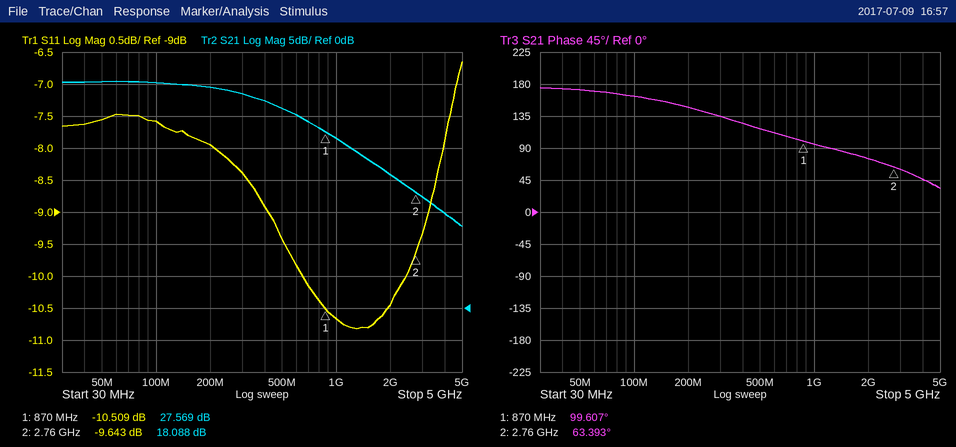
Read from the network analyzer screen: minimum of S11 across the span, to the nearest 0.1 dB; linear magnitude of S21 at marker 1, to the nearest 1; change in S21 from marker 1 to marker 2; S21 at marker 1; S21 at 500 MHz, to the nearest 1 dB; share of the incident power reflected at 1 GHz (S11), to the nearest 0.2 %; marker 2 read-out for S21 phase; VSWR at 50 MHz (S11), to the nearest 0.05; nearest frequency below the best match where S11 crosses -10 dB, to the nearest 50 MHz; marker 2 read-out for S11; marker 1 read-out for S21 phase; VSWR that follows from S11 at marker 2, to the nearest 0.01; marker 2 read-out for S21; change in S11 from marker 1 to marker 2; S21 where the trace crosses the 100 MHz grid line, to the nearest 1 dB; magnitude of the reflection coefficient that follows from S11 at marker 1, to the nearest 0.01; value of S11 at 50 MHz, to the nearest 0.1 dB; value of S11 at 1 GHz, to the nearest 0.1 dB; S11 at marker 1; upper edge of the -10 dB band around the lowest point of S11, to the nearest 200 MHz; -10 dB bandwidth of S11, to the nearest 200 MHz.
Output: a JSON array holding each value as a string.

["-10.8 dB", "24", "-9.481 dB", "27.569 dB", "31 dB", "8.6 %", "63.393°", "2.45", "650 MHz", "-9.643 dB", "99.607°", "1.98", "18.088 dB", "0.866 dB", "35 dB", "0.30", "-7.6 dB", "-10.7 dB", "-10.509 dB", "2.4 GHz", "1.8 GHz"]
